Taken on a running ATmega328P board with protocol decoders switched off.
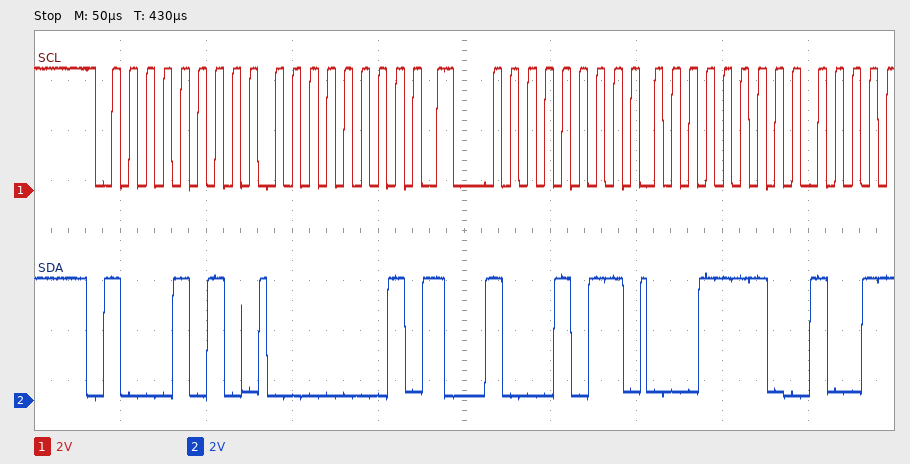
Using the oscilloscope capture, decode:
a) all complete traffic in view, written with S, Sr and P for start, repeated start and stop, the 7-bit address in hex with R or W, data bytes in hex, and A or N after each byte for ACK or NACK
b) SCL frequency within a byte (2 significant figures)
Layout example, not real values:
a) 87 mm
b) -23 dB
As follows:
a) S 45W A 01 A Sr 45R A 1E A
b) 100 kHz
